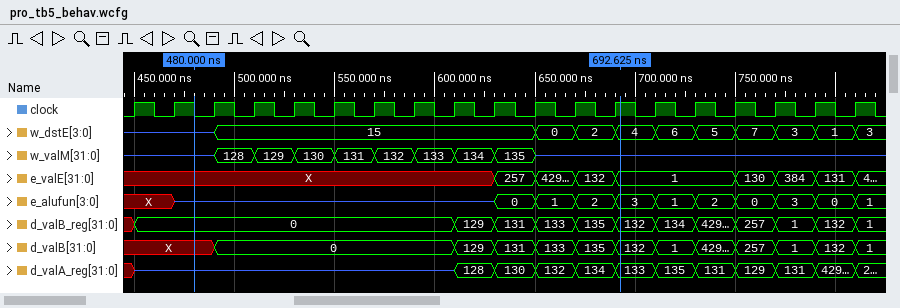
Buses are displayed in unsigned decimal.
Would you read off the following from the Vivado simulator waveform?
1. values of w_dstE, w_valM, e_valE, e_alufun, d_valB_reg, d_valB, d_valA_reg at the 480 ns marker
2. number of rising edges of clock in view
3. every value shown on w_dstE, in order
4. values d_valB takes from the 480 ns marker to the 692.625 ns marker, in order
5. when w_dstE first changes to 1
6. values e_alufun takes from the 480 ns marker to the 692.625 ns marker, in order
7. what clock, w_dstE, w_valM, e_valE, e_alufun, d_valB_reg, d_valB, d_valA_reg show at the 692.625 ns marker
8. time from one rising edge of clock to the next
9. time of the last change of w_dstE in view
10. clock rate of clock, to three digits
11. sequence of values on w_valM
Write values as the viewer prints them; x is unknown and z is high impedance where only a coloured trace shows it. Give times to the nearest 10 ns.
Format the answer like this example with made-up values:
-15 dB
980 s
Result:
w_dstE=z, w_valM=z, e_valE=X, e_alufun=z, d_valB_reg=0, d_valB=X, d_valA_reg=z
19
z, 15, 0, 2, 4, 6, 5, 7, 3, 1, 3
X, 0, 129, 131, 133, 135, 132
790 ns
z, 0, 1, 2, 3
clock=1, w_dstE=4, w_valM=z, e_valE=1, e_alufun=3, d_valB_reg=132, d_valB=132, d_valA_reg=133
20 ns
810 ns
50.0 MHz
z, 128, 129, 130, 131, 132, 133, 134, 135, z
